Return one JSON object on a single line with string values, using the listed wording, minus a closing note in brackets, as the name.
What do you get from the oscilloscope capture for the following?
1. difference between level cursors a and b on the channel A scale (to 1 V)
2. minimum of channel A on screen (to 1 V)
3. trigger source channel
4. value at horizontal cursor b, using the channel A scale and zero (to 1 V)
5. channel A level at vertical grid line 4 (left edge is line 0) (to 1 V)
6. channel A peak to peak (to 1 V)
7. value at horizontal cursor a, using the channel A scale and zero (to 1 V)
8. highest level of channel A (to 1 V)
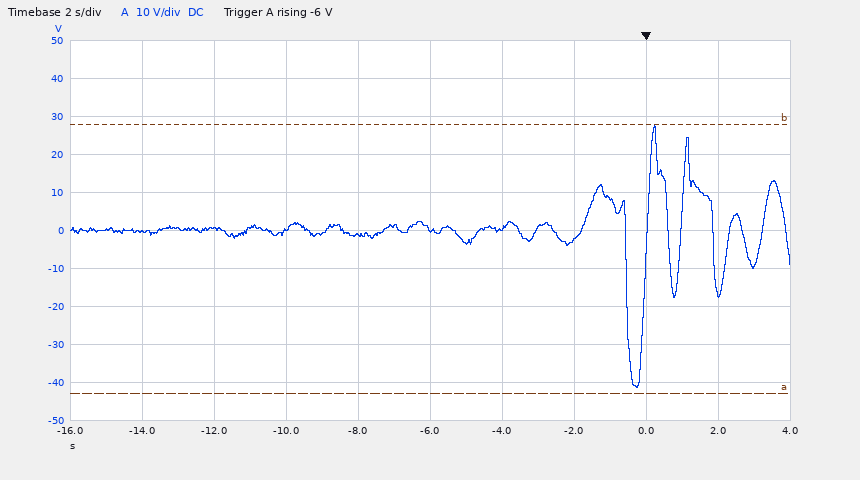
{"difference between level cursors a and b on the channel A scale": "71 V", "minimum of channel A on screen": "-41 V", "trigger source channel": "channel A", "value at horizontal cursor b, using the channel A scale and zero": "28 V", "channel A level at vertical grid line 4 (left edge is line 0)": "-1 V", "channel A peak to peak": "69 V", "value at horizontal cursor a, using the channel A scale and zero": "-43 V", "highest level of channel A": "28 V"}
